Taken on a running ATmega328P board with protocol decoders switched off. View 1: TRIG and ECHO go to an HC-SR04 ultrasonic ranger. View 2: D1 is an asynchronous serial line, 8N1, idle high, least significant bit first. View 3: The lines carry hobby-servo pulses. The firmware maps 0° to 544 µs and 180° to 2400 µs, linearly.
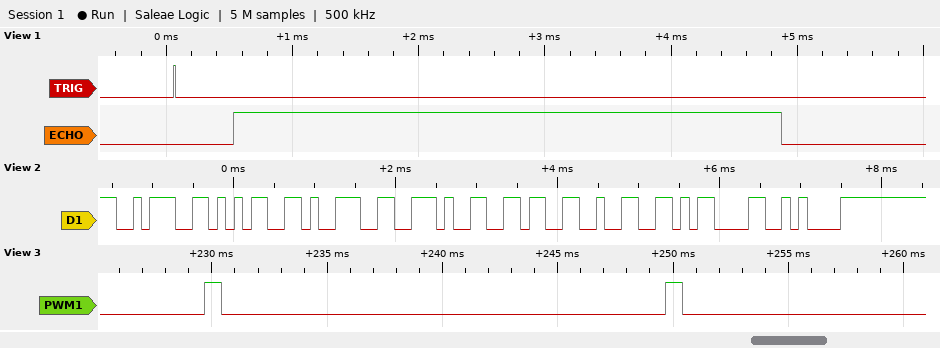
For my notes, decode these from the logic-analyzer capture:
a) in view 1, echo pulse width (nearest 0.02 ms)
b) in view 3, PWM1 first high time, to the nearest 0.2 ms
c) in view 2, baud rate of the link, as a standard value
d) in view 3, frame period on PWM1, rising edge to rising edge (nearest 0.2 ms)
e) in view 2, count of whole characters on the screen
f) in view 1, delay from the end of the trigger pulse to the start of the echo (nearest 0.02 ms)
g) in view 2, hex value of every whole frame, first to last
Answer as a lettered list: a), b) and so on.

a) 4.34 ms
b) 0.8 ms
c) 9600 baud
d) 20.0 ms
e) 8
f) 0.46 ms
g) 0x3A 0x35 0x39 0x2E 0x36 0x32 0x0D 0x0A
